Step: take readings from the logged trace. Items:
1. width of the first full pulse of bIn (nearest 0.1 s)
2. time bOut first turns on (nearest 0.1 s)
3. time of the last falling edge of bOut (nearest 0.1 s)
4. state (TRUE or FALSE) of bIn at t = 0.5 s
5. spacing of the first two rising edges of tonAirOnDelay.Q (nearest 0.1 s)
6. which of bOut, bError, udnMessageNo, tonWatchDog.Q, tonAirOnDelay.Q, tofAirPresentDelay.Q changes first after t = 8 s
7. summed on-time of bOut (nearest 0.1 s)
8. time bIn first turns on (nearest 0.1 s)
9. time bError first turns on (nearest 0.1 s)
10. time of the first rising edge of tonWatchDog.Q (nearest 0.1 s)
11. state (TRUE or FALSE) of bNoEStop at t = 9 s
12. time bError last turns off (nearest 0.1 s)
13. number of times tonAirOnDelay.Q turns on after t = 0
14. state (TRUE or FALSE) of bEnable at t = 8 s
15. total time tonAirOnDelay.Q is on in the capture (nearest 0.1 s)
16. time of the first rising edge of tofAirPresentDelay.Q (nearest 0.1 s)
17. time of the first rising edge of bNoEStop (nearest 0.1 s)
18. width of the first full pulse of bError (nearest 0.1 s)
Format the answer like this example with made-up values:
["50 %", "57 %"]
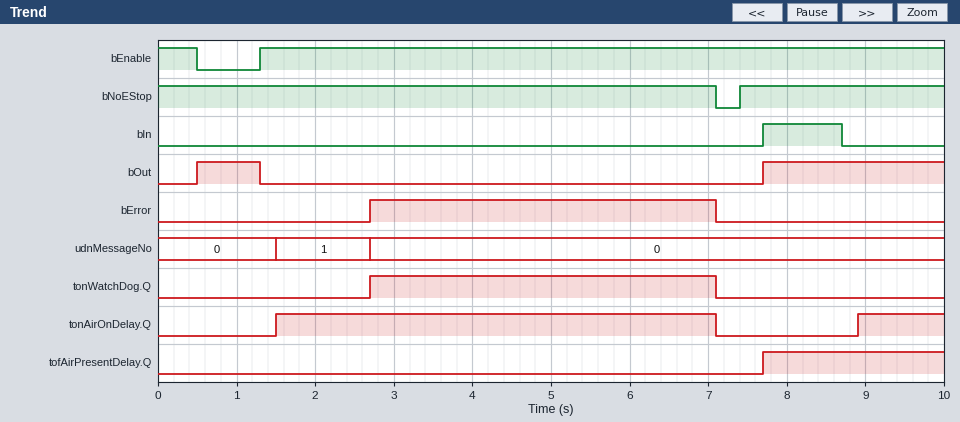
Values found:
["1.0 s", "0.5 s", "1.3 s", "FALSE", "7.4 s", "tonAirOnDelay.Q", "3.1 s", "7.7 s", "2.7 s", "2.7 s", "TRUE", "7.1 s", "2", "TRUE", "6.7 s", "7.7 s", "7.4 s", "4.4 s"]
